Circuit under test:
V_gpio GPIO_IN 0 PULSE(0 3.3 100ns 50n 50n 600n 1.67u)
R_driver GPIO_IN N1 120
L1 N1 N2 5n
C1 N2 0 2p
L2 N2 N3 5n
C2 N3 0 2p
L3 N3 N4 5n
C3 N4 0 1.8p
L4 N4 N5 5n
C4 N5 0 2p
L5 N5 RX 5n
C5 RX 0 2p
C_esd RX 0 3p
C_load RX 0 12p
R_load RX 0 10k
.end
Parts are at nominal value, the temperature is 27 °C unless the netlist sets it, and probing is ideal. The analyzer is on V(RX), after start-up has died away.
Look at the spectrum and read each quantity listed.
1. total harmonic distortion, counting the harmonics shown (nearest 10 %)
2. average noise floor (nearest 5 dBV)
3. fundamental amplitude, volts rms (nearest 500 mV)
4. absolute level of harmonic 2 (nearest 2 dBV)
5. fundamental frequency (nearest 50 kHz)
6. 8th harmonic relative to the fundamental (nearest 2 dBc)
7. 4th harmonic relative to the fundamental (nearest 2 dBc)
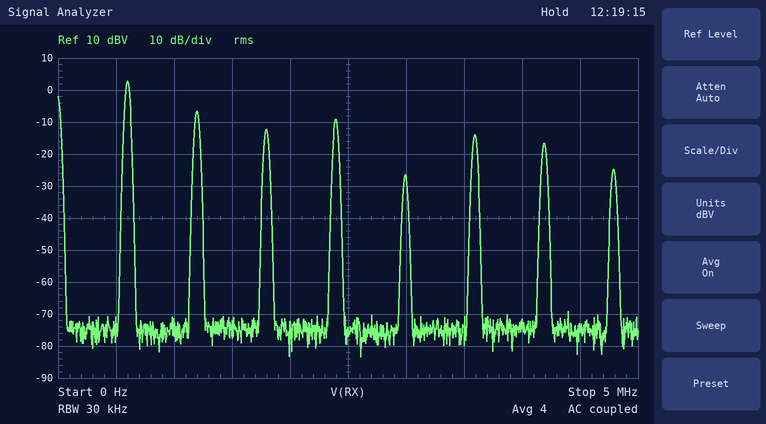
50 %
-75 dBV
1.5 V
-6 dBV
600 kHz
-28 dBc
-12 dBc
